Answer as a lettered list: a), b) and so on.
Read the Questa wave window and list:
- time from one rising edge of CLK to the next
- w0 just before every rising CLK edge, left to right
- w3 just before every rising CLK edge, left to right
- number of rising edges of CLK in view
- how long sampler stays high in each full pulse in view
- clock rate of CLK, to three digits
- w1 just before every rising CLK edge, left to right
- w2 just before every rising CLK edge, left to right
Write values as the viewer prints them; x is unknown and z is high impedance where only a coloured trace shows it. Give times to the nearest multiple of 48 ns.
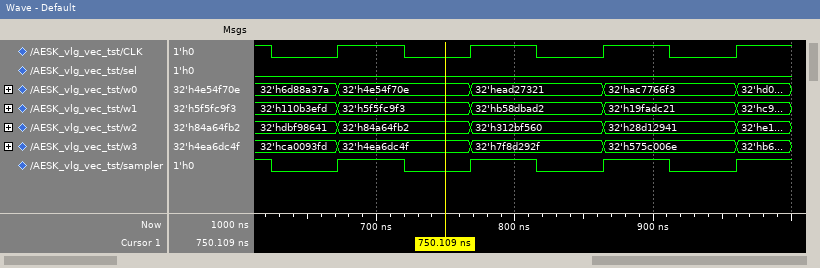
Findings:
a) 96 ns
b) 32'h6d88a37a, 32'h4e54f70e, 32'head27321, 32'hac7766f3
c) 32'hca0093fd, 32'h4ea6dc4f, 32'h7f8d292f, 32'h575c006e
d) 4
e) 48 ns, 48 ns, 48 ns
f) 10.4 MHz
g) 32'h110b3efd, 32'h5f5fc9f3, 32'hb58dbad2, 32'h19fadc21
h) 32'hdbf98641, 32'h84a64fb2, 32'h312bf560, 32'h28d12941
